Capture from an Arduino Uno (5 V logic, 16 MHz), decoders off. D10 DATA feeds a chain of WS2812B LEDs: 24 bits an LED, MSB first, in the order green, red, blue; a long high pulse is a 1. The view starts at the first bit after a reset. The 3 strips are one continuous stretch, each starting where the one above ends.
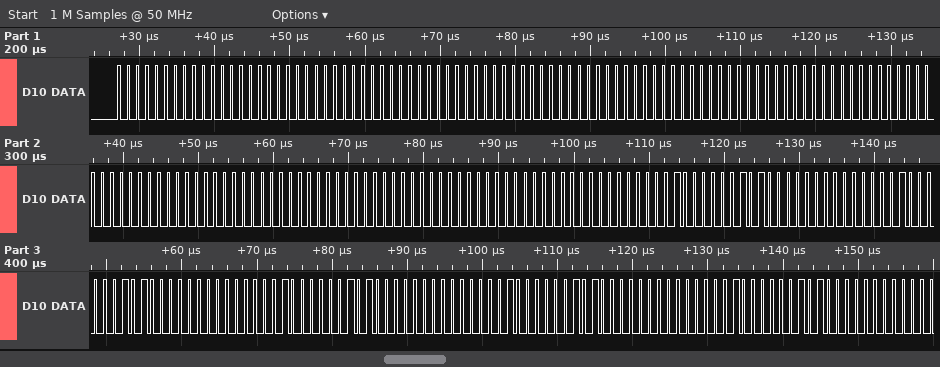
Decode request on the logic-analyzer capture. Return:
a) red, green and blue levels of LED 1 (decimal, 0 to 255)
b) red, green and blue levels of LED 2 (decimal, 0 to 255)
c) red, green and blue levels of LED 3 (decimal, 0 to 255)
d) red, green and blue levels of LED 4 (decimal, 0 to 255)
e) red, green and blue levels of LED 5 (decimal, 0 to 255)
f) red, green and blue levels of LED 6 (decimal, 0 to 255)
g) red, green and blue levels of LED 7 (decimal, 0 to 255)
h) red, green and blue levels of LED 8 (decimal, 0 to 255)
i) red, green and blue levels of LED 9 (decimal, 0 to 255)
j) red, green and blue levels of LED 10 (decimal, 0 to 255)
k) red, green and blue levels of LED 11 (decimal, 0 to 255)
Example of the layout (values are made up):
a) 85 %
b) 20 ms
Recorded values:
a) 0, 0, 0
b) 0, 0, 0
c) 0, 0, 0
d) 0, 0, 0
e) 0, 0, 0
f) 0, 0, 0
g) 10, 4, 0
h) 10, 4, 0
i) 10, 4, 0
j) 10, 4, 0
k) 10, 4, 0
